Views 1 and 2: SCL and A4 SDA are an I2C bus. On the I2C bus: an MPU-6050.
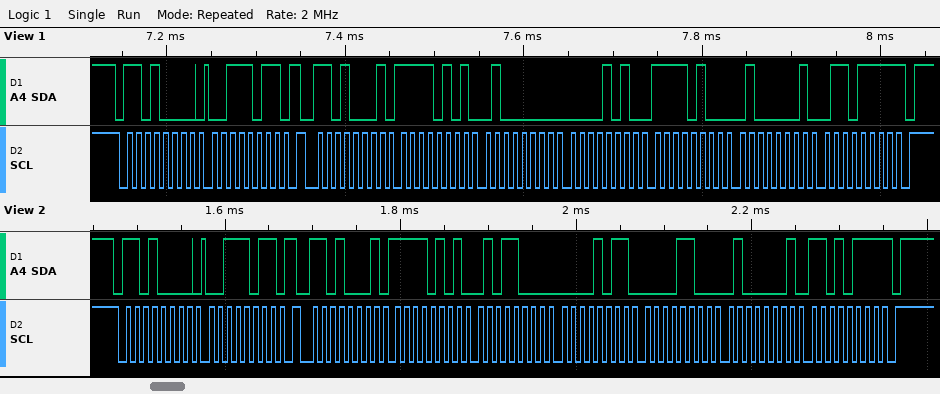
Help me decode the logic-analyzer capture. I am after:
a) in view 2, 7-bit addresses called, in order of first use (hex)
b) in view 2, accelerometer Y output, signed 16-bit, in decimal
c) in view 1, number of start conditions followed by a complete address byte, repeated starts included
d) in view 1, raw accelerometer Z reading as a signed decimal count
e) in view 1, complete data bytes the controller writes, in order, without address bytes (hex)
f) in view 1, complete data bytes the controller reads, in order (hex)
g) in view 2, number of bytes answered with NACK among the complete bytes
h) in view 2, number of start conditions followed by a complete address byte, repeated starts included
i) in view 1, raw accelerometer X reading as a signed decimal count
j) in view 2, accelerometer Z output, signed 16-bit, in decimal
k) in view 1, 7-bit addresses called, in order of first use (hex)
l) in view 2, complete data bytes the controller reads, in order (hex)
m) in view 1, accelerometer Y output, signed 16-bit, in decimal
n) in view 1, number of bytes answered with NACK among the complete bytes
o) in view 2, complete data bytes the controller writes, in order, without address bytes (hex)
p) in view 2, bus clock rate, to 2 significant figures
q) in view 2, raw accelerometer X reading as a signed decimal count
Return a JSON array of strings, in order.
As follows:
["0x68", "2828", "2", "16751", "3B", "F5 40 0A F4 41 6F", "1", "2", "-2752", "16855", "0x68", "F5 58 0B 0C 41 D7", "2804", "1", "3B", "100 kHz", "-2728"]
